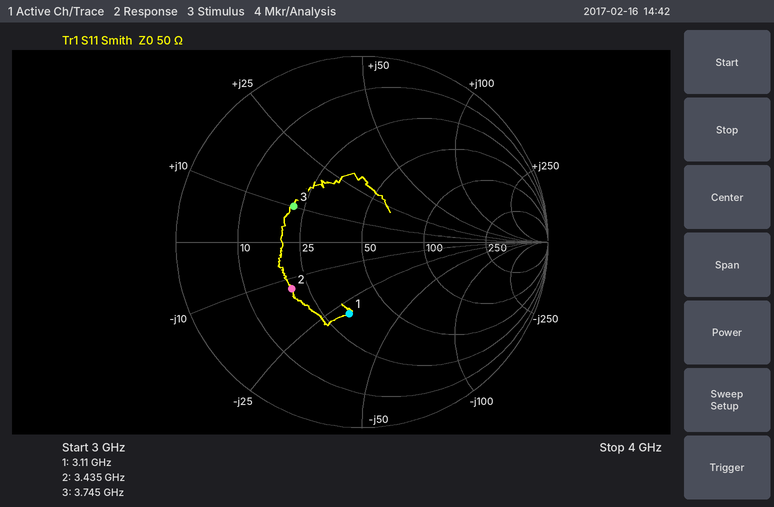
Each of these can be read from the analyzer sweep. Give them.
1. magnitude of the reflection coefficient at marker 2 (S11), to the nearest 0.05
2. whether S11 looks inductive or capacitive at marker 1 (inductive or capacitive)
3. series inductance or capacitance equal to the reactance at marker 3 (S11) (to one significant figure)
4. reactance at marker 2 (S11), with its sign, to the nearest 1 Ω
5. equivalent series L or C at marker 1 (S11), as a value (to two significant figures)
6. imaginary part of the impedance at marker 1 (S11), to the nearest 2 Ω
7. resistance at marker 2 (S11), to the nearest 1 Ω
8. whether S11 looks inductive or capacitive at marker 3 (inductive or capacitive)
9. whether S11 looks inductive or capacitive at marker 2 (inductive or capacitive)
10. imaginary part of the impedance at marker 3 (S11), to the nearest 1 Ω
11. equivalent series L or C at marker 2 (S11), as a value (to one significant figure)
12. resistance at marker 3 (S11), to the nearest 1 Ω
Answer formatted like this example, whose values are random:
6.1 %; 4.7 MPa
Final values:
0.45; capacitive; 400 pH; -13 Ω; 1.7 pF; -30 Ω; 20 Ω; inductive; capacitive; +10 Ω; 4 pF; 22 Ω
